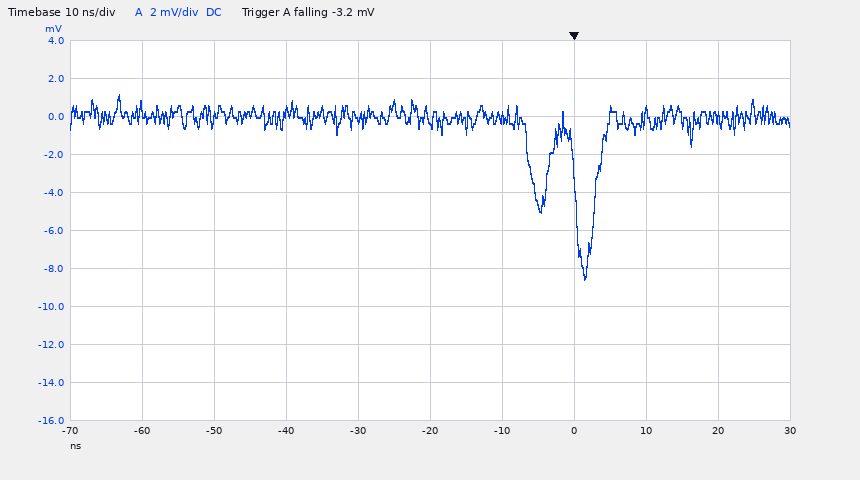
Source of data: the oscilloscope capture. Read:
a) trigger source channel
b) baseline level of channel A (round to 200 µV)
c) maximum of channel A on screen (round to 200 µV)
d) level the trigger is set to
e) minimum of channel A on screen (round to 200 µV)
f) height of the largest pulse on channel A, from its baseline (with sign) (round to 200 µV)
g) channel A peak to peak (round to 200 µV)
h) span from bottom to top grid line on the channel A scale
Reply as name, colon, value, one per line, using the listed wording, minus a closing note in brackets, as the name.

trigger source channel: channel A
baseline level of channel A: 0.0 mV
maximum of channel A on screen: 1.2 mV
level the trigger is set to: -3.2 mV
minimum of channel A on screen: -8.6 mV
height of the largest pulse on channel A, from its baseline (with sign): -8.6 mV
channel A peak to peak: 9.8 mV
span from bottom to top grid line on the channel A scale: 20 mV
